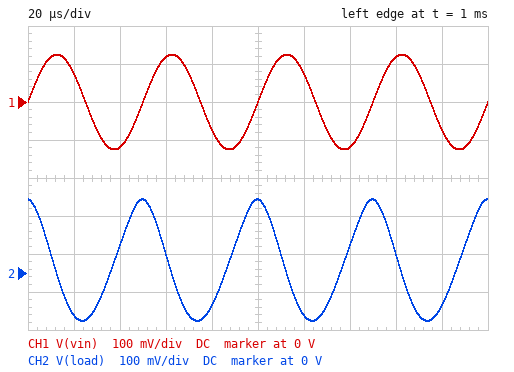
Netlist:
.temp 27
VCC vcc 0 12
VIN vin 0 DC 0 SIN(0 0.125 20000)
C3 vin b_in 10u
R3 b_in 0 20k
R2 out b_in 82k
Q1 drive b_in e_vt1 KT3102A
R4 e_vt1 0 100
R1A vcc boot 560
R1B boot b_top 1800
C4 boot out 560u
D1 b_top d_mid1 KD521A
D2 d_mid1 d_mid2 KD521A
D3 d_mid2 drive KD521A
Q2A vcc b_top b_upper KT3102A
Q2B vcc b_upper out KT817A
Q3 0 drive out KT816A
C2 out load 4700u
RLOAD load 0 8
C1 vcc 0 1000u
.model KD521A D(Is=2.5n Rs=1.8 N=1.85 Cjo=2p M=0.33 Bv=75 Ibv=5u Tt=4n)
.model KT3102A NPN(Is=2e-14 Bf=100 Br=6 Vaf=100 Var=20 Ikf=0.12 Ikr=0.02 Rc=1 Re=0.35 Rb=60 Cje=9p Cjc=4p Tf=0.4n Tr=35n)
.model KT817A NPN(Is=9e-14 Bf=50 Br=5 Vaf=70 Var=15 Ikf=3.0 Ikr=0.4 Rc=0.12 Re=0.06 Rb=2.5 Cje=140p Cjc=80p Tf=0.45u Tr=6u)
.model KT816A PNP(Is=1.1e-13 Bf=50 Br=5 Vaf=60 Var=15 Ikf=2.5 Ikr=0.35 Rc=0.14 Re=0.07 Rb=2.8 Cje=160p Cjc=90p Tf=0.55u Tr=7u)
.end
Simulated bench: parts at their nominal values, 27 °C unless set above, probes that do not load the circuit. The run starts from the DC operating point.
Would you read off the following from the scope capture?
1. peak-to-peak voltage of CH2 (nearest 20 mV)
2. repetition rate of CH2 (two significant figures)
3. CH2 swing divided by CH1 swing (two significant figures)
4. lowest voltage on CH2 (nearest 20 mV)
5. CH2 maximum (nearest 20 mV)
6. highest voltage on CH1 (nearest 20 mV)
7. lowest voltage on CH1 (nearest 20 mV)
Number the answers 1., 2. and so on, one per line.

1. 320 mV
2. 20 kHz
3. 1.3
4. -120 mV
5. 200 mV
6. 120 mV
7. -120 mV
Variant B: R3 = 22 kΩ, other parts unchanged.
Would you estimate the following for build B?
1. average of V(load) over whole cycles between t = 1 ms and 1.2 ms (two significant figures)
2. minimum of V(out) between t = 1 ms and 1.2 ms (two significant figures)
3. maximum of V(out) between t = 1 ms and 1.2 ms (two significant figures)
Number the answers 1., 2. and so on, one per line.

1. 20 mV
2. 6.0 V
3. 6.3 V
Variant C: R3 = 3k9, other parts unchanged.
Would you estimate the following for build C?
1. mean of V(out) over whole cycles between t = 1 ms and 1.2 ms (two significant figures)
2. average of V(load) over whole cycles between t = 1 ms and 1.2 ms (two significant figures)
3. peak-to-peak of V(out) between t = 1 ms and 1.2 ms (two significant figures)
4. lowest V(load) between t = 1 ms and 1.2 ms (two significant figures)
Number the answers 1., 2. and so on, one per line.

1. 11 V
2. -5.3 mV
3. 17 mV
4. -17 mV
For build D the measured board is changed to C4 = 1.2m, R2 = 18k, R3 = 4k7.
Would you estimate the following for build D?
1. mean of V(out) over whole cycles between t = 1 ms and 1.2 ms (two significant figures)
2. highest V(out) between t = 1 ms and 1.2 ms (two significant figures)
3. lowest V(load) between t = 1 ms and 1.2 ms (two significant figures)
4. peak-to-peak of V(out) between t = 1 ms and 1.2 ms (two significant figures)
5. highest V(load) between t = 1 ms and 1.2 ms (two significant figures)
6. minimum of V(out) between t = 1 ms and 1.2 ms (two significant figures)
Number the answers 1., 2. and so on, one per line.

1. 5.2 V
2. 5.3 V
3. -140 mV
4. 310 mV
5. 170 mV
6. 5.0 V
